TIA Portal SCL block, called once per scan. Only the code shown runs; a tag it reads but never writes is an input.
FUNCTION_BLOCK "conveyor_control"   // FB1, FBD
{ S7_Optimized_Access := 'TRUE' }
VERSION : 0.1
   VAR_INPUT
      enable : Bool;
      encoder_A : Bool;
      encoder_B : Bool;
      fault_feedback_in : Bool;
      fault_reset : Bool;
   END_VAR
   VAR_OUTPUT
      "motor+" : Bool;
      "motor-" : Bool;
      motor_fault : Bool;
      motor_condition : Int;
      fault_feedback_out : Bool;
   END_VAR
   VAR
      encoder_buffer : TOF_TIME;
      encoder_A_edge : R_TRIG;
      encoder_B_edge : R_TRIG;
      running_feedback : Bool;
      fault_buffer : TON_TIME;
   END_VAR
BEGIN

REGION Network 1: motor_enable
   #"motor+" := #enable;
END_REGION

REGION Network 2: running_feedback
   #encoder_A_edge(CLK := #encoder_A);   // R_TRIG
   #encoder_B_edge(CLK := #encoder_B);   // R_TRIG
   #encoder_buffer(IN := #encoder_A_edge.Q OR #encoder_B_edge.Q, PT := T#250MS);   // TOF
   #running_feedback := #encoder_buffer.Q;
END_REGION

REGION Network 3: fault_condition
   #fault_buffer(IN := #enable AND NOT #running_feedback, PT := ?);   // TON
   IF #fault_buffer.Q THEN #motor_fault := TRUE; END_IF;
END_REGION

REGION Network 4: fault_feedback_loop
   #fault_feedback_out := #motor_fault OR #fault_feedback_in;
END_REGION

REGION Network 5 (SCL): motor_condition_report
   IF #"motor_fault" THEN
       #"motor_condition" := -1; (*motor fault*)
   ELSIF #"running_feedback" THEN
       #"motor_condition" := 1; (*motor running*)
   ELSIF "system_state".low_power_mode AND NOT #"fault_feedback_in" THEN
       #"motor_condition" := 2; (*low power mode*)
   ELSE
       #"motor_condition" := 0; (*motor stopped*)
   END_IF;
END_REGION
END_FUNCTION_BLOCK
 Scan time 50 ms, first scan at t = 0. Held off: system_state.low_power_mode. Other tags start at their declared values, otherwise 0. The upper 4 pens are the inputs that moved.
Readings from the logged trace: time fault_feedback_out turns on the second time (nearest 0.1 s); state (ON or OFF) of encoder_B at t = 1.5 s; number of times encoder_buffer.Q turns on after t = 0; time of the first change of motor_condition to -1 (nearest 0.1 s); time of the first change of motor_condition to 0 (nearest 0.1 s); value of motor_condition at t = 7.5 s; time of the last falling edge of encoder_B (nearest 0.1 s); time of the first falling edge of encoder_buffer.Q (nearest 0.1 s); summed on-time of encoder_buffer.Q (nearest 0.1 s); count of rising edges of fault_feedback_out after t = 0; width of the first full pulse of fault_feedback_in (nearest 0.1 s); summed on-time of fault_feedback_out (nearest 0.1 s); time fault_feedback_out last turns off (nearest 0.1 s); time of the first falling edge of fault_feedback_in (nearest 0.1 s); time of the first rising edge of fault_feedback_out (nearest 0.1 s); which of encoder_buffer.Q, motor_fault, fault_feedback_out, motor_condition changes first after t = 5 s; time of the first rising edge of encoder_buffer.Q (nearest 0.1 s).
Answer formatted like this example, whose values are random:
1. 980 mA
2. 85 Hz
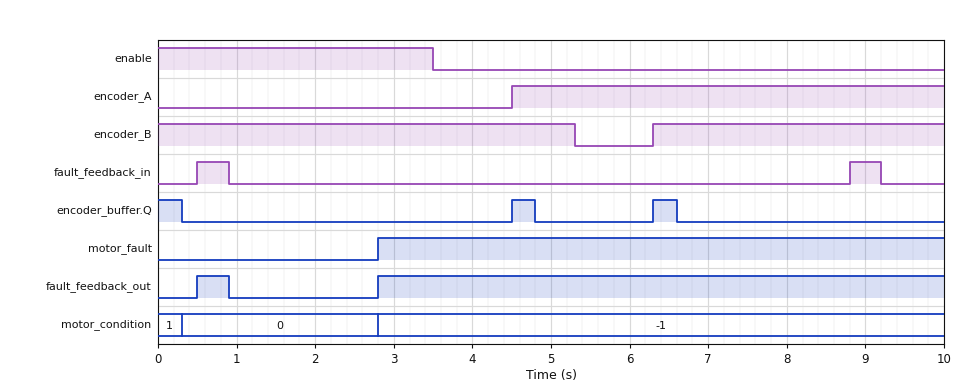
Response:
1. 2.8 s
2. ON
3. 2
4. 2.8 s
5. 0.3 s
6. -1
7. 5.3 s
8. 0.3 s
9. 0.9 s
10. 2
11. 0.4 s
12. 7.6 s
13. 0.9 s
14. 0.9 s
15. 0.5 s
16. encoder_buffer.Q
17. 4.5 s
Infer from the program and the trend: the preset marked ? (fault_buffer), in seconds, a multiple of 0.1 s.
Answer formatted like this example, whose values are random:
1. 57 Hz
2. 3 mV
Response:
1. 2.5 s
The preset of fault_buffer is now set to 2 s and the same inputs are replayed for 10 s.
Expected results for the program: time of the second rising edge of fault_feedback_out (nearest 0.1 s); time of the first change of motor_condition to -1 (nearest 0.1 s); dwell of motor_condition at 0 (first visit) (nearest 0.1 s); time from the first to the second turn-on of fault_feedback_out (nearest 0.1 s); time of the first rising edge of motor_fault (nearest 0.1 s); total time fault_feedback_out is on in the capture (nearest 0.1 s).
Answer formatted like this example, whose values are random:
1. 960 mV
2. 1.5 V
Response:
1. 2.3 s
2. 2.3 s
3. 2.0 s
4. 1.8 s
5. 2.3 s
6. 8.1 s
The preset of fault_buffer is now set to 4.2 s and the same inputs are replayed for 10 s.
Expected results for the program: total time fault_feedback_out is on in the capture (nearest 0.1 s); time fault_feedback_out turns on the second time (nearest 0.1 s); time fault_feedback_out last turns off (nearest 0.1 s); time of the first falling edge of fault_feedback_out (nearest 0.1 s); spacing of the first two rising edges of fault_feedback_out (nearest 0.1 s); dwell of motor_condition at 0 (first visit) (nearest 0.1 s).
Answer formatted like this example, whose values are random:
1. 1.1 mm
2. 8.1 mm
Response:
1. 0.8 s
2. 8.8 s
3. 9.2 s
4. 0.9 s
5. 8.3 s
6. 4.2 s
